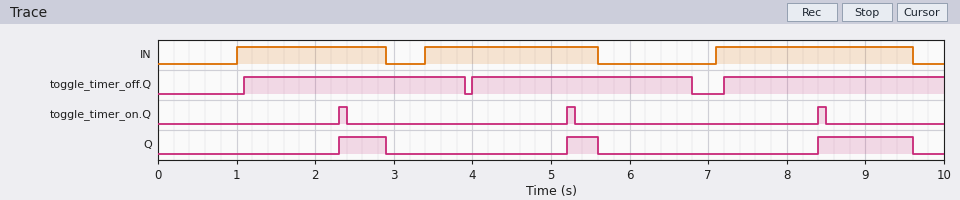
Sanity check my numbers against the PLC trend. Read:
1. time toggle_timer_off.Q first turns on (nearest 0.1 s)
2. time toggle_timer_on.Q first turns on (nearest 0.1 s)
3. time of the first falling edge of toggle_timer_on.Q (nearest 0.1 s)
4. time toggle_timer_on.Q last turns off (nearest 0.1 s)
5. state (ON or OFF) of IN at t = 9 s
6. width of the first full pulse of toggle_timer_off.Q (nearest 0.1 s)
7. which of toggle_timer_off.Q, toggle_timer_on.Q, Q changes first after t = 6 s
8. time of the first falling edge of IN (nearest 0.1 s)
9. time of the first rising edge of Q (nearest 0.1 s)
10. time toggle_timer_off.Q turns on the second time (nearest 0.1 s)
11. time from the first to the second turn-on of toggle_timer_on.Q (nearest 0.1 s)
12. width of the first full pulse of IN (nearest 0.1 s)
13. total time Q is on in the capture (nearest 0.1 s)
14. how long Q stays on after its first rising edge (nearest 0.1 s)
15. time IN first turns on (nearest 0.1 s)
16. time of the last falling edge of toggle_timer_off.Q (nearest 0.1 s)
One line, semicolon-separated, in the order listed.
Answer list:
1.1 s; 2.3 s; 2.4 s; 8.5 s; ON; 2.8 s; toggle_timer_off.Q; 2.9 s; 2.3 s; 4.0 s; 2.9 s; 1.9 s; 2.2 s; 0.6 s; 1.0 s; 6.8 s
